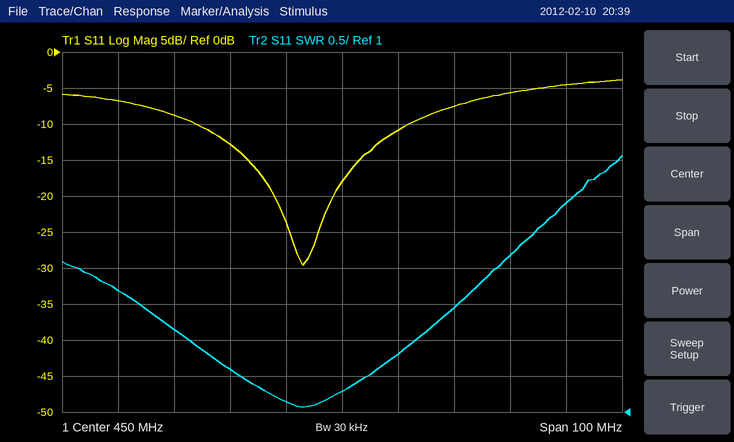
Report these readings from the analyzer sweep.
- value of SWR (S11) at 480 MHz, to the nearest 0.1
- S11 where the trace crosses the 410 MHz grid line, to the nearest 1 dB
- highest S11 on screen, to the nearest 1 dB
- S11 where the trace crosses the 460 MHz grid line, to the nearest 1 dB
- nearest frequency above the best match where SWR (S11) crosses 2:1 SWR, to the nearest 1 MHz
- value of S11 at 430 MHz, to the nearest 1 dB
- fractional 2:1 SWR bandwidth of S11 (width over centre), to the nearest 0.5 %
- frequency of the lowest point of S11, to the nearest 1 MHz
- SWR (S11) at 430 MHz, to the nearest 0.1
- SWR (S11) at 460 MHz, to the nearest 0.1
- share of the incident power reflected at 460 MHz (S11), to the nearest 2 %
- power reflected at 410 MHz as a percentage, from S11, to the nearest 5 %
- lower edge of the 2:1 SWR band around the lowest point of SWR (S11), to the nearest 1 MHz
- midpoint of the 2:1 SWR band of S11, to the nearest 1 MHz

3.2
-7 dB
-4 dB
-11 dB
463 MHz
-13 dB
9.0 %
443 MHz
1.6
1.8
8 %
20 %
423 MHz
443 MHz
